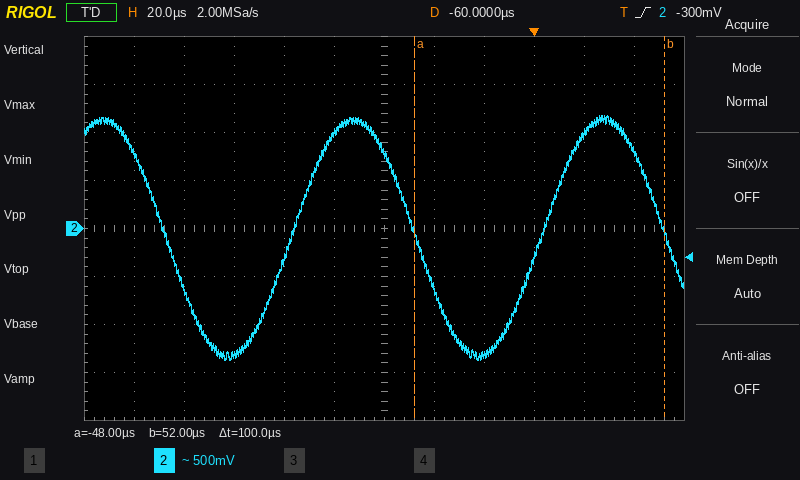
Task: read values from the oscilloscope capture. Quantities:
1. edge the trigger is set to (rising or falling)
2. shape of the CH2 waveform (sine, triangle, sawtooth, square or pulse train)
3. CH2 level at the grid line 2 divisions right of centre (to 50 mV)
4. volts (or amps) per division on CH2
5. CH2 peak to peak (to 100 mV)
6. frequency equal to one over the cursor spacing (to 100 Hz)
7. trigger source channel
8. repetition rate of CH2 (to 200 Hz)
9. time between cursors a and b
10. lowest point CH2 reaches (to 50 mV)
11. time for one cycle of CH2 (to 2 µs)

rising
sine
-1.30 V
500 mV
2.50 V
10.0 kHz
CH2
10.0 kHz
100 µs
-1.35 V
100 µs
